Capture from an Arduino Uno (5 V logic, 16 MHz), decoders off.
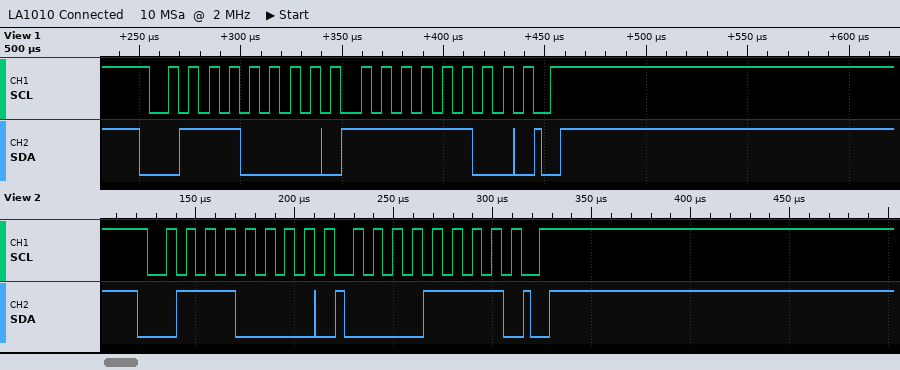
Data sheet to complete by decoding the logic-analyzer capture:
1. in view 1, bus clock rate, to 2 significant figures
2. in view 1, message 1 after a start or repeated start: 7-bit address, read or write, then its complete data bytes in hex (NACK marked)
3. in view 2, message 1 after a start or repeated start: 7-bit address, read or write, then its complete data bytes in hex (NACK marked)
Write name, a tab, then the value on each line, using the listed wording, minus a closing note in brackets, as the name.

in view 1, bus clock rate, to 2 significant figures	100 kHz
in view 1, message 1 after a start or repeated start: 7-bit address, read or write, then its complete data bytes in hex	0x38 write: FC
in view 2, message 1 after a start or repeated start: 7-bit address, read or write, then its complete data bytes in hex	0x38 write: 0F
